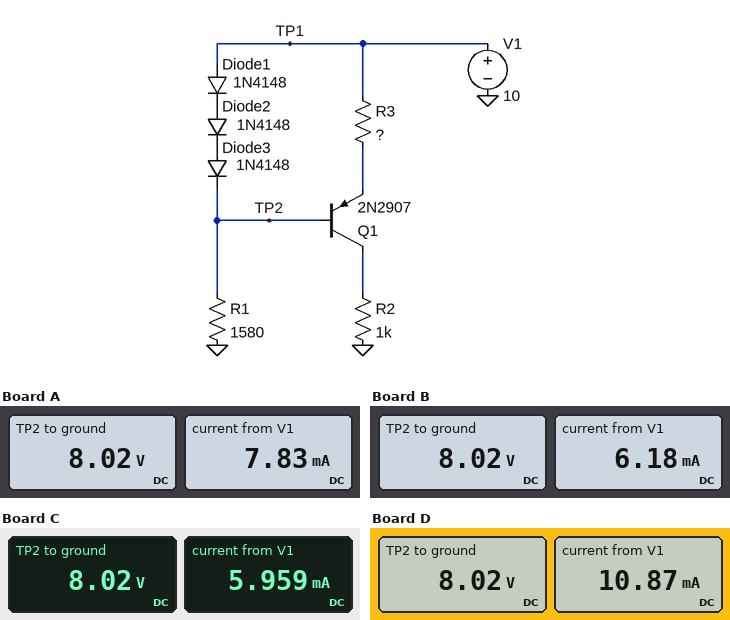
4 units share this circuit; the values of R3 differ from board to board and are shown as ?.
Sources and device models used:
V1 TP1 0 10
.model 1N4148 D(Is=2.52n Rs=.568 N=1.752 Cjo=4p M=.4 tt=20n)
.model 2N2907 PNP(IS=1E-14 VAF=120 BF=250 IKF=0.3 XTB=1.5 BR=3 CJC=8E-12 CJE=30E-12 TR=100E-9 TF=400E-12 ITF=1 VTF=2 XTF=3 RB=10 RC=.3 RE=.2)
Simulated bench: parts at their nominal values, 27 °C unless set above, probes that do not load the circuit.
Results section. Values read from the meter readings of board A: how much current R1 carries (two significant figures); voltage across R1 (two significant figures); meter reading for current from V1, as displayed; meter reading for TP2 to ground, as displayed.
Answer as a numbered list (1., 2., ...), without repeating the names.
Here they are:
1. 5.1 mA
2. 8.0 V
3. 7.83 mA
4. 8.02 V
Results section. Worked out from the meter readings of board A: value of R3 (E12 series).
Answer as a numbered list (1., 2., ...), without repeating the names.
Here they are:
1. 470 Ω
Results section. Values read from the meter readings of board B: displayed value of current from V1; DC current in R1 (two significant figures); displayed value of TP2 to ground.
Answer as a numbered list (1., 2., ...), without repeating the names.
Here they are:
1. 6.18 mA
2. 5.1 mA
3. 8.02 V
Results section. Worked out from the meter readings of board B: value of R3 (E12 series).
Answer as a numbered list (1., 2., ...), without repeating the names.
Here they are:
1. 1.2 kΩ
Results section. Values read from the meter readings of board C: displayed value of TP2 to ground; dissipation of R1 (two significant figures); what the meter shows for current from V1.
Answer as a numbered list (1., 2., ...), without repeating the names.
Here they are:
1. 8.02 V
2. 41 mW
3. 5.959 mA
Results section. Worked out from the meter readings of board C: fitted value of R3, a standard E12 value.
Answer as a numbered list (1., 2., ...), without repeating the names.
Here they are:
1. 1.5 kΩ
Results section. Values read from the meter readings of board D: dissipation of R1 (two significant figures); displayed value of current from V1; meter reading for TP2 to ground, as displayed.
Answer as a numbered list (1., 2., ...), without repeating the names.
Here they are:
1. 41 mW
2. 10.87 mA
3. 8.02 V
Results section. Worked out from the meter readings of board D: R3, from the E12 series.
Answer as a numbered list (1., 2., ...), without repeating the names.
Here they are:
1. 220 Ω
